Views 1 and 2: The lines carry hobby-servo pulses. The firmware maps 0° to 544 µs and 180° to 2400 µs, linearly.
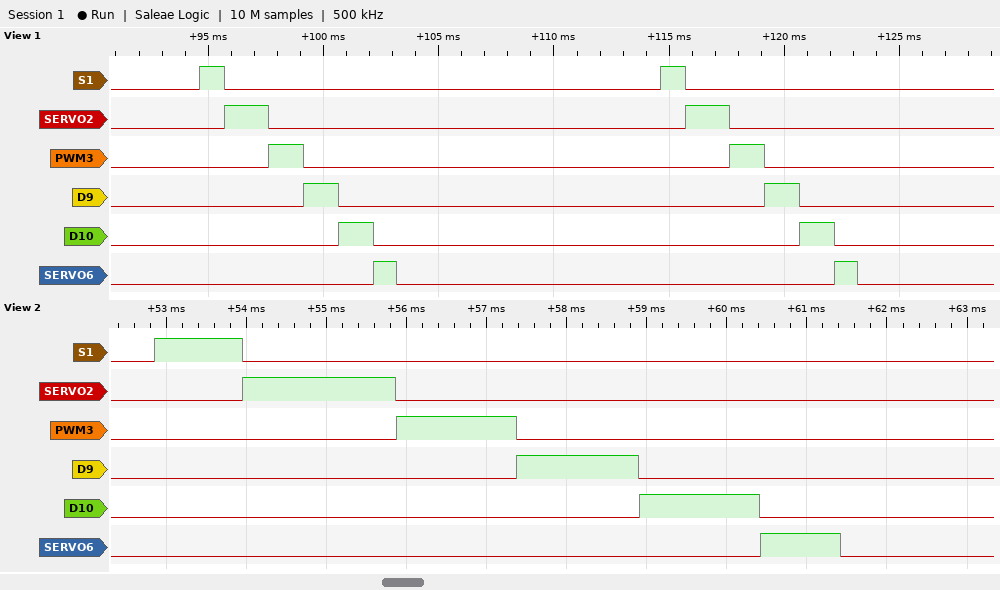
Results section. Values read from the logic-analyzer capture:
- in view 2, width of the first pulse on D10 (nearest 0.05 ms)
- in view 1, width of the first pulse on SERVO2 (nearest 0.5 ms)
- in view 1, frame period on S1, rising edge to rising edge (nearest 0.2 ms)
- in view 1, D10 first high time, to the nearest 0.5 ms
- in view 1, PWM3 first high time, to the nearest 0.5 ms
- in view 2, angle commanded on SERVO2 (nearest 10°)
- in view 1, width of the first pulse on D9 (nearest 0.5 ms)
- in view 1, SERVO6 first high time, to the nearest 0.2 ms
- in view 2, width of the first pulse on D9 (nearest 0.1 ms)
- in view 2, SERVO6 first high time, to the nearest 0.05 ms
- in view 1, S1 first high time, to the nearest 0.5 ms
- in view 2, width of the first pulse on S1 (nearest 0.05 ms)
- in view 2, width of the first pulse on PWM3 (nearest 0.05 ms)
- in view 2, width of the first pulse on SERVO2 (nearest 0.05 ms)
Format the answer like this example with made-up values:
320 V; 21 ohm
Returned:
1.50 ms; 2.0 ms; 20.0 ms; 1.5 ms; 1.5 ms; 130°; 1.5 ms; 1.0 ms; 1.5 ms; 1.00 ms; 1.0 ms; 1.10 ms; 1.50 ms; 1.90 ms
